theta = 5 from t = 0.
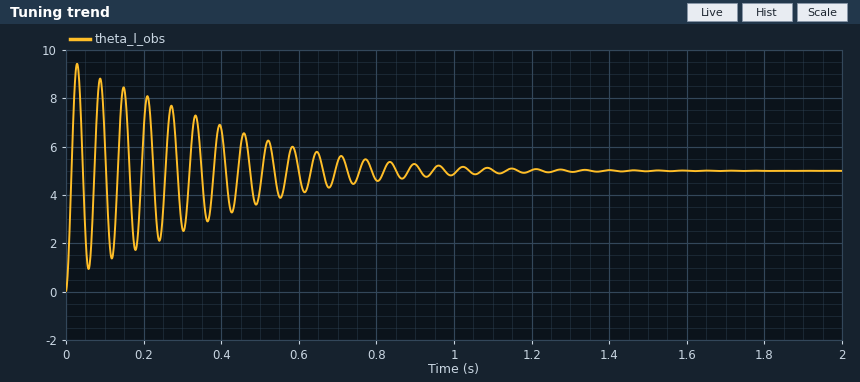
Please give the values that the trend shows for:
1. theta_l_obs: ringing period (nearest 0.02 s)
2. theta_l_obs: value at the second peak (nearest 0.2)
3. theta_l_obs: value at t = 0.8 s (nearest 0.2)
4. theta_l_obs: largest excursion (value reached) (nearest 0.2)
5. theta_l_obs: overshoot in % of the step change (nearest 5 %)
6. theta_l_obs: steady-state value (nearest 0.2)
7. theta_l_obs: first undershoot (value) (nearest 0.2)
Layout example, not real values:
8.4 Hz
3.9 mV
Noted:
0.06 s
8.8
4.6
9.4
90 %
5.0
1.0
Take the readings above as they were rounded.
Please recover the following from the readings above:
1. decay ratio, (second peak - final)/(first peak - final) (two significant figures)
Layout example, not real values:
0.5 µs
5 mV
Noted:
0.86
